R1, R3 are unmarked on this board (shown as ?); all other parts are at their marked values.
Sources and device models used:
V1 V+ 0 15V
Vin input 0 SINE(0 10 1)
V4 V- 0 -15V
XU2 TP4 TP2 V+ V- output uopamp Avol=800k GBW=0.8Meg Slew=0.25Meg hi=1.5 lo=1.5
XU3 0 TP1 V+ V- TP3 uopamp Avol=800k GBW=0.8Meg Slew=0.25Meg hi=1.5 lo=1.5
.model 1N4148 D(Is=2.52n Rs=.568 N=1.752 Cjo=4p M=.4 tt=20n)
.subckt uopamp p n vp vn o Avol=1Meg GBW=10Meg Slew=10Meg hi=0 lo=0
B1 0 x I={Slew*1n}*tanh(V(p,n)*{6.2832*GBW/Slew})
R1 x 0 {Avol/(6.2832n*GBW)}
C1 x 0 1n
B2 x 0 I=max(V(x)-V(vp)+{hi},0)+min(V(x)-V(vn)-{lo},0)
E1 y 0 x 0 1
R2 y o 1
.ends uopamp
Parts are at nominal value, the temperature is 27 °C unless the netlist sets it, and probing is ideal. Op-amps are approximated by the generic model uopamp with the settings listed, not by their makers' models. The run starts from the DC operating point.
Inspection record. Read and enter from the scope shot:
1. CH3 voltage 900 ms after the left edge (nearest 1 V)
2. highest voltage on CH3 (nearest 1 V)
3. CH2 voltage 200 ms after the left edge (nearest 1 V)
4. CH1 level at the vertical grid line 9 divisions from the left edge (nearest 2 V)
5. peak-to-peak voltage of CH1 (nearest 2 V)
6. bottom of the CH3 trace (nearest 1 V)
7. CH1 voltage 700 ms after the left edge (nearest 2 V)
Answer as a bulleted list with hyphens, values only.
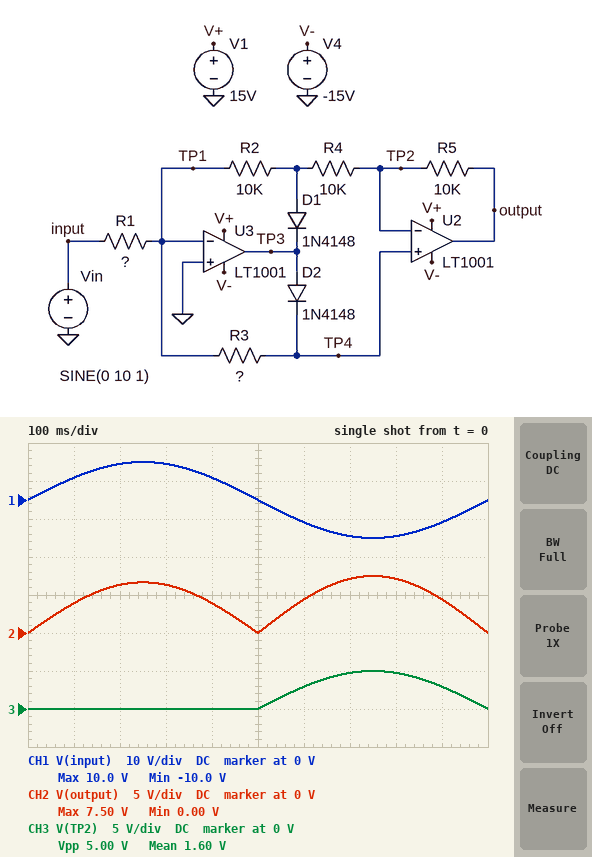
- 3 V
- 5 V
- 6 V
- -6 V
- 20 V
- 0 V
- -10 V
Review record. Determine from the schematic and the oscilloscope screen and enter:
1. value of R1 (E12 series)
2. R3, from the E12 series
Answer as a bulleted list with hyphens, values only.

- 15 kΩ
- 12 kΩ
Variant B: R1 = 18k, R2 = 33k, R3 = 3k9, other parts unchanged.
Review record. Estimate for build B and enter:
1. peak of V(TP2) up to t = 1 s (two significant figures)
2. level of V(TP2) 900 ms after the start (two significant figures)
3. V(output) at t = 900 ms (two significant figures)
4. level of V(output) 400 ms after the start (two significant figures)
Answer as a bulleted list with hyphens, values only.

- 2.0 V
- 1.2 V
- 1.4 V
- 11 V
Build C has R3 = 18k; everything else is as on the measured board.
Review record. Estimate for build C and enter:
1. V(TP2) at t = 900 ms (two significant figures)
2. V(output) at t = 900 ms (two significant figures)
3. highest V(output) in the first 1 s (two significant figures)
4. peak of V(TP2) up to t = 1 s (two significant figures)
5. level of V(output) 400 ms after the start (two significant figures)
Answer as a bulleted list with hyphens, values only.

- 3.7 V
- 5.6 V
- 9.5 V
- 6.3 V
- 3.9 V
